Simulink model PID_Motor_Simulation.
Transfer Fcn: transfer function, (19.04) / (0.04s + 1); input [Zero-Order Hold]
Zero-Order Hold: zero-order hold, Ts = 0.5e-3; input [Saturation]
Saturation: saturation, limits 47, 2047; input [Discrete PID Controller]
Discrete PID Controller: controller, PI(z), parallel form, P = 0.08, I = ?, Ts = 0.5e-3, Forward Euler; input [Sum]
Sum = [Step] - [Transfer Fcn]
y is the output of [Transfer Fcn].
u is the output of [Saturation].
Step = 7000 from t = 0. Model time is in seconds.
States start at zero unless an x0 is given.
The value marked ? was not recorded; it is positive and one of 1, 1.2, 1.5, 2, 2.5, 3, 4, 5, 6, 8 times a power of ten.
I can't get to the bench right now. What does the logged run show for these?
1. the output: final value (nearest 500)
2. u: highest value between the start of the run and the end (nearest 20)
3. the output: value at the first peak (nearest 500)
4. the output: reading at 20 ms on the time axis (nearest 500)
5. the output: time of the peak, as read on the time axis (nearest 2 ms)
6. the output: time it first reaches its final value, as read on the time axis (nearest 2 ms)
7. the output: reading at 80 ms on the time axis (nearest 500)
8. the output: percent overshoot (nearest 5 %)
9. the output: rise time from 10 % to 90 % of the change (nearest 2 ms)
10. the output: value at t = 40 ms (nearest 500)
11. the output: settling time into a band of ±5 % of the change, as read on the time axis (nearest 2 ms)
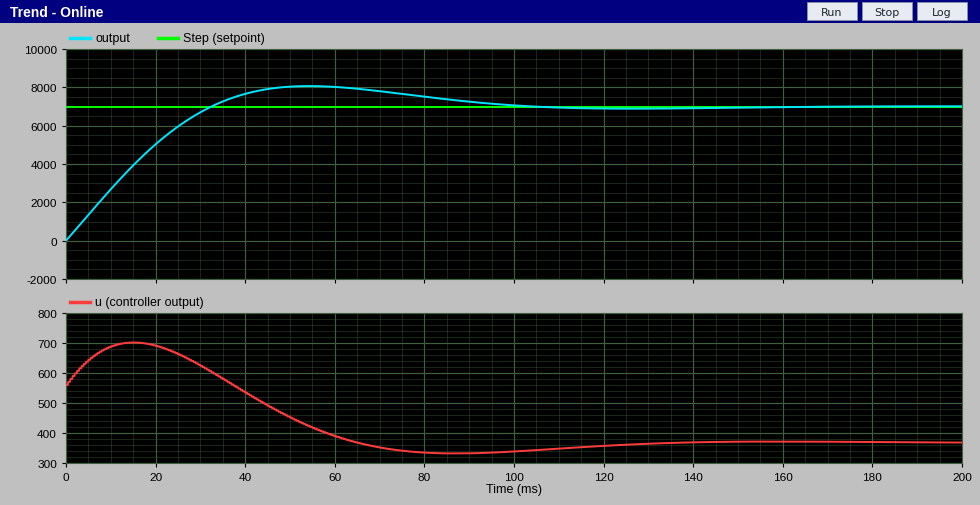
7000
700
8000
5000
54 ms
32 ms
7500
15 %
24 ms
7500
86 ms
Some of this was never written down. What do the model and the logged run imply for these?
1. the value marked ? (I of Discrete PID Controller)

6
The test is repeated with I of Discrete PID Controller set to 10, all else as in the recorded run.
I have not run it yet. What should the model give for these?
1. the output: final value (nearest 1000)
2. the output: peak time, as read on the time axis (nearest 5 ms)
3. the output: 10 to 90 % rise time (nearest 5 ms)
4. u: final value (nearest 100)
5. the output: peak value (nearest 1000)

7000
40 ms
20 ms
400
9000
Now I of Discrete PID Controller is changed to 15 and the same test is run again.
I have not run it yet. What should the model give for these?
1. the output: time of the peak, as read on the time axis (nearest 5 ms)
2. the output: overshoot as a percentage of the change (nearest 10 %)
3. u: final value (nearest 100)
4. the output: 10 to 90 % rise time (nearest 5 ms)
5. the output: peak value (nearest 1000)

35 ms
30 %
400
15 ms
9000
